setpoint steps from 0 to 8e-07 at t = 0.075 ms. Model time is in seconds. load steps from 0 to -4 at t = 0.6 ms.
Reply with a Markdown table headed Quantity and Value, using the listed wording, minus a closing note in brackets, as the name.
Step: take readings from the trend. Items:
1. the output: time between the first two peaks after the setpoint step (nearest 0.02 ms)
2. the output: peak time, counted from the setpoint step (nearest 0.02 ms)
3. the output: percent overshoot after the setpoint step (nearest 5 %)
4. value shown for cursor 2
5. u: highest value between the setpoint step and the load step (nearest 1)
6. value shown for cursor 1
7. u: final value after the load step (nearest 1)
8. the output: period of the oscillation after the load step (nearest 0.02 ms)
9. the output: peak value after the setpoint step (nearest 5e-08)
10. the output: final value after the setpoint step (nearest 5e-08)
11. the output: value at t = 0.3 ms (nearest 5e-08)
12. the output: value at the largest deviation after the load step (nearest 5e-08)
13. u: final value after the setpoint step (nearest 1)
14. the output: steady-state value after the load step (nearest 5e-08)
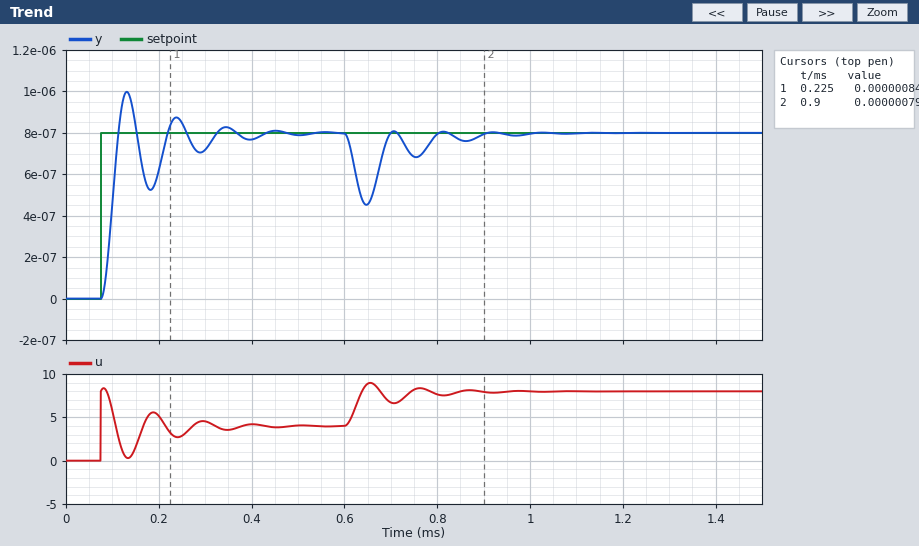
| Quantity | Value |
|---|---|
| the output: time between the first two peaks after the setpoint step | 0.10 ms |
| the output: peak time, counted from the setpoint step | 0.06 ms |
| the output: percent overshoot after the setpoint step | 25 % |
| value shown for cursor 2 | 0.000000795 |
| u: highest value between the setpoint step and the load step | 8 |
| value shown for cursor 1 | 0.000000840 |
| u: final value after the load step | 8 |
| the output: period of the oscillation after the load step | 0.10 ms |
| the output: peak value after the setpoint step | 0.00000100 |
| the output: final value after the setpoint step | 0.00000080 |
| the output: value at t = 0.3 ms | 0.00000070 |
| the output: value at the largest deviation after the load step | 0.00000045 |
| u: final value after the setpoint step | 4 |
| the output: steady-state value after the load step | 0.00000080 |
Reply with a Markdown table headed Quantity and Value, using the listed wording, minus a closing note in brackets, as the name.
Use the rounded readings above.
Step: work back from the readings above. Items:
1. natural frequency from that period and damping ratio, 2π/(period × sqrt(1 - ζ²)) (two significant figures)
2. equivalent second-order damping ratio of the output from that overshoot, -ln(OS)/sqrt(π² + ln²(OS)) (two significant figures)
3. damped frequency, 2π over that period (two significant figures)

| Quantity | Value |
|---|---|
| natural frequency from that period and damping ratio, 2π/(period × sqrt(1 - ζ²)) | 69 rad/ms |
| equivalent second-order damping ratio of the output from that overshoot, -ln(OS)/sqrt(π² + ln²(OS)) | 0.40 |
| damped frequency, 2π over that period | 63 rad/ms |
